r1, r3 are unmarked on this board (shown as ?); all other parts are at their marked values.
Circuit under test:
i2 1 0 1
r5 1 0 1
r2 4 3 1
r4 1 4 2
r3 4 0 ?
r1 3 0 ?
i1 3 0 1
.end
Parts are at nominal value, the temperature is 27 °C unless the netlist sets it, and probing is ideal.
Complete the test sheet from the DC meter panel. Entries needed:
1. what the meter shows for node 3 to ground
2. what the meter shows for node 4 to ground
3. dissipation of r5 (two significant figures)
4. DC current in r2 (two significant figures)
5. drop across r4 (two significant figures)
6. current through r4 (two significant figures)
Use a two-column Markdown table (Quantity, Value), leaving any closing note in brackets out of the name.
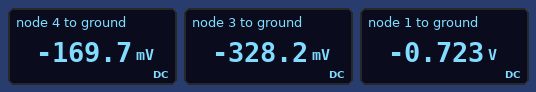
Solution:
| Quantity | Value |
|---|---|
| what the meter shows for node 3 to ground | -328.2 mV |
| what the meter shows for node 4 to ground | -169.7 mV |
| dissipation of r5 | 520 mW |
| DC current in r2 | 160 mA |
| drop across r4 | 550 mV |
| current through r4 | 280 mA |
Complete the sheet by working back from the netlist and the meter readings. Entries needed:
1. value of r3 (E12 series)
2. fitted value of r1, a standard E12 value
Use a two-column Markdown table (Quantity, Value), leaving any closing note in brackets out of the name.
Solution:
| Quantity | Value |
|---|---|
| value of r3 | 0.39 Ω |
| fitted value of r1, a standard E12 value | 0.39 Ω |
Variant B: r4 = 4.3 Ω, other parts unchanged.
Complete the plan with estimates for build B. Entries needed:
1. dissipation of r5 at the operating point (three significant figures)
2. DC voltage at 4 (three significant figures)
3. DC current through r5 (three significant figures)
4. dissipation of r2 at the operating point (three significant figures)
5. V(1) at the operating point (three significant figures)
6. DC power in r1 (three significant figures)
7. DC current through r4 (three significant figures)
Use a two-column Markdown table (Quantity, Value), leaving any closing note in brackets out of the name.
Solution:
| Quantity | Value |
|---|---|
| dissipation of r5 at the operating point | 700 mW |
| DC voltage at 4 | -135 mV |
| DC current through r5 | 837 mA |
| dissipation of r2 at the operating point | 33.6 mW |
| V(1) at the operating point | -837 mV |
| DC power in r1 | 260 mW |
| DC current through r4 | 163 mA |
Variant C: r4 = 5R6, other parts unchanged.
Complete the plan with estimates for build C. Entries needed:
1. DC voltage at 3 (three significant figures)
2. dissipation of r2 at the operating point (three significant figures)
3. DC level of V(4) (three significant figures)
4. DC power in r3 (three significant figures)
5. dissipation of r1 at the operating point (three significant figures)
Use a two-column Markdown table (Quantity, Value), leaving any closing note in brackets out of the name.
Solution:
| Quantity | Value |
|---|---|
| DC voltage at 3 | -316 mV |
| dissipation of r2 at the operating point | 36.1 mW |
| DC level of V(4) | -126 mV |
| DC power in r3 | 40.6 mW |
| dissipation of r1 at the operating point | 256 mW |
